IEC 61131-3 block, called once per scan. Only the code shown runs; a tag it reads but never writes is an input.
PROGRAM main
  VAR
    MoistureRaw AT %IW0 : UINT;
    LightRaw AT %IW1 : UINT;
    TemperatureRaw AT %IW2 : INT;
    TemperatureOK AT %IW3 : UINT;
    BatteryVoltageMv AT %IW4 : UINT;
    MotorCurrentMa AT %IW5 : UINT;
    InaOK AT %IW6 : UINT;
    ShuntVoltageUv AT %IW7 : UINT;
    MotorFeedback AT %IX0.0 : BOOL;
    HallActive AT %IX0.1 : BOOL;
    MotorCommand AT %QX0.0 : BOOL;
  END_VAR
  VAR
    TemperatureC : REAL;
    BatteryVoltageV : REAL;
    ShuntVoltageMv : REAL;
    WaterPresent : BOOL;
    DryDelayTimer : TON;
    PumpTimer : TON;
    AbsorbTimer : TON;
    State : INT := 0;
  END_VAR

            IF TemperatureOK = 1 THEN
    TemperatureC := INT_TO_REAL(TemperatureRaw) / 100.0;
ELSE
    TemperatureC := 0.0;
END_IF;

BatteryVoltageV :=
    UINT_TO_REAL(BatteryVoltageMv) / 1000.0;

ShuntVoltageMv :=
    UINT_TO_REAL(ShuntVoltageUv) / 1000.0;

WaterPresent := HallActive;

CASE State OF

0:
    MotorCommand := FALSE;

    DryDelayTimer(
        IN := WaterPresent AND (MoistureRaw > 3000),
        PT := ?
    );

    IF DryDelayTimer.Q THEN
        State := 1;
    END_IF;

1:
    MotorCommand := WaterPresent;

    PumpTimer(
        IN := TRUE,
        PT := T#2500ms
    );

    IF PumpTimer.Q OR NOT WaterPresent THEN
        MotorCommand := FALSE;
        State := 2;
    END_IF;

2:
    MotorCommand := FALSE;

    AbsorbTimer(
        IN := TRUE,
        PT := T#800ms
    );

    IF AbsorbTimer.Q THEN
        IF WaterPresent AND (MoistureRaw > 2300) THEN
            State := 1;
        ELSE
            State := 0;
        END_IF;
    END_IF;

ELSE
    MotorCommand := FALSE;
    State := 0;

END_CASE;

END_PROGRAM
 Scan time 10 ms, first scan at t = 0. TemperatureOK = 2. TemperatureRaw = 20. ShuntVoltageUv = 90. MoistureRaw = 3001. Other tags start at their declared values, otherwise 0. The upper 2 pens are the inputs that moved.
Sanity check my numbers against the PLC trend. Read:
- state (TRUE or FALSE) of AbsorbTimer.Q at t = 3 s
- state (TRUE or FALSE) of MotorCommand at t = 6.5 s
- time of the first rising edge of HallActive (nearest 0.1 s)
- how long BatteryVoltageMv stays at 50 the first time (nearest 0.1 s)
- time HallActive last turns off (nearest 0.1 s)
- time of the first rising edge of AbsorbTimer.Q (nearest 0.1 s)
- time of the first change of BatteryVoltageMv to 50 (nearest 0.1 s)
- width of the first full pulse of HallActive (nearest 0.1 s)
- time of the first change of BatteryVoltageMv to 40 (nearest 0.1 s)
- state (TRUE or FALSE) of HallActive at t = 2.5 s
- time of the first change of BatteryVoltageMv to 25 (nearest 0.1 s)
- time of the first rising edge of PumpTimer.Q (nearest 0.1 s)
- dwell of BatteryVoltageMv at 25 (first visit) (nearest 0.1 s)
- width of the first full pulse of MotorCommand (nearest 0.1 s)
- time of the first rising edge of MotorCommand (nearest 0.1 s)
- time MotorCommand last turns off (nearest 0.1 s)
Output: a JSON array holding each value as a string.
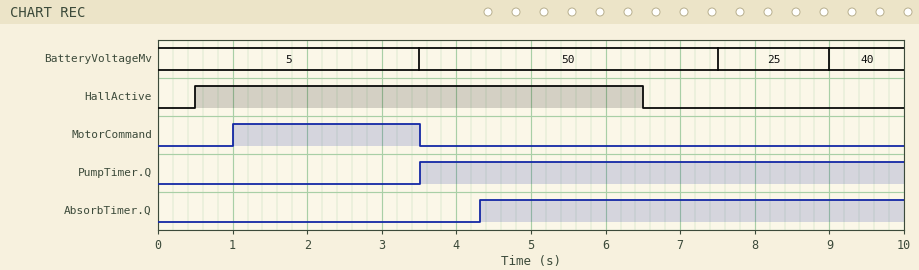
["FALSE", "FALSE", "0.5 s", "4.0 s", "6.5 s", "4.3 s", "3.5 s", "6.0 s", "9.0 s", "TRUE", "7.5 s", "3.5 s", "1.5 s", "2.5 s", "1.0 s", "3.5 s"]
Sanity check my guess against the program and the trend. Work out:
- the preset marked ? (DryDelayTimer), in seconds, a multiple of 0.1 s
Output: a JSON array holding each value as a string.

["0.5 s"]
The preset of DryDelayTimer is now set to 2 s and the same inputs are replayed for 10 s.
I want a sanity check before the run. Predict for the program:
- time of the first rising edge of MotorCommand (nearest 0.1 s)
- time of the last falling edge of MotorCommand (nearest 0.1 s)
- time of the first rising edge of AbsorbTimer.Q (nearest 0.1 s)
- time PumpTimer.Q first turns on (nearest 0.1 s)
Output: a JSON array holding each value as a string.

["2.5 s", "5.0 s", "5.8 s", "5.0 s"]
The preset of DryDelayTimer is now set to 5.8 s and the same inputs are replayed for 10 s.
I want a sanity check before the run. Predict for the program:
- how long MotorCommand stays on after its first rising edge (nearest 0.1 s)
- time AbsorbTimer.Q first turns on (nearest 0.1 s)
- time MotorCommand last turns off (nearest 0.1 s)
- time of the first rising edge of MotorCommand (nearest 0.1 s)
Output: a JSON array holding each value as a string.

["0.2 s", "7.3 s", "6.5 s", "6.3 s"]
